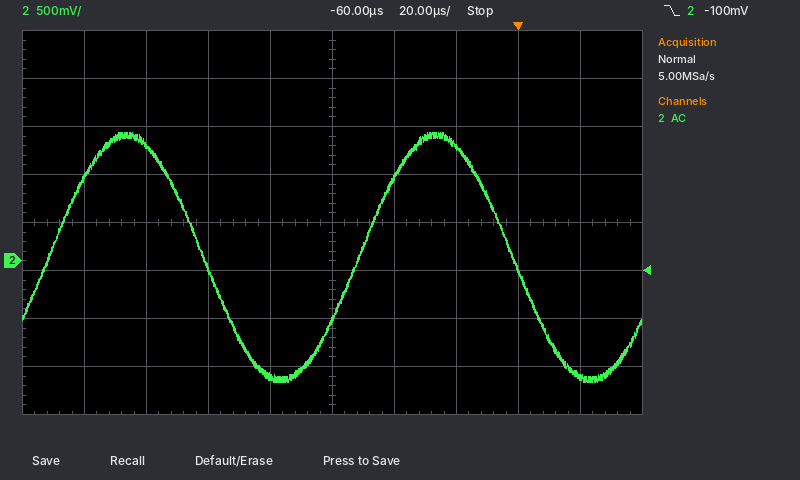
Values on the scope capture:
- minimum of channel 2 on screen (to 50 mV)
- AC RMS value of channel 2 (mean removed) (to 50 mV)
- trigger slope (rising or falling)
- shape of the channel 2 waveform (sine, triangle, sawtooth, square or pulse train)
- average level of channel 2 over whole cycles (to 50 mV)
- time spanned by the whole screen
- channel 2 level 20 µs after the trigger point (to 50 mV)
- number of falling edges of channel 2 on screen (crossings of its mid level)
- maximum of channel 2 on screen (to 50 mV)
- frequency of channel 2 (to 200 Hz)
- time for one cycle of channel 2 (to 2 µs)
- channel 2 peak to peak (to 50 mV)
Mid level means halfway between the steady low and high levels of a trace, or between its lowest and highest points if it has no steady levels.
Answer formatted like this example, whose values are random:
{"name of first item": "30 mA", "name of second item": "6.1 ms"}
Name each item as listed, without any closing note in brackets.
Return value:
{"minimum of channel 2 on screen": "-1.25 V", "AC RMS value of channel 2 (mean removed)": "900 mV", "trigger slope": "falling", "shape of the channel 2 waveform": "sine", "average level of channel 2 over whole cycles": "50 mV", "time spanned by the whole screen": "200 µs", "channel 2 level 20 µs after the trigger point": "-1.20 V", "number of falling edges of channel 2 on screen": "2", "maximum of channel 2 on screen": "1.35 V", "frequency of channel 2": "10.0 kHz", "time for one cycle of channel 2": "100 µs", "channel 2 peak to peak": "2.60 V"}
